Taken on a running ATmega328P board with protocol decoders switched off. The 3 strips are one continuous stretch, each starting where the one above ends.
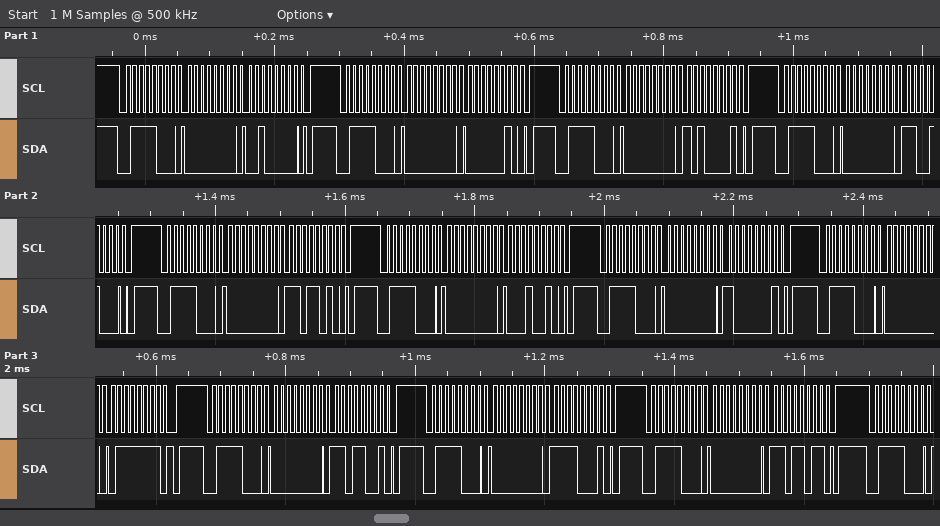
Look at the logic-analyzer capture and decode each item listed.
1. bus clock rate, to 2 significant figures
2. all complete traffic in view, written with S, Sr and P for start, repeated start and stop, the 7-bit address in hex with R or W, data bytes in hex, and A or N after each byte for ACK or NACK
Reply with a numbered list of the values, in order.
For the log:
1. 100 kHz
2. S 3CW A 00 A 20 A P S 3CW A 00 A 02 A P S 3CW A 00 A A1 A P S 3CW A 00 A C8 A P S 3CW A 00 A DA A P S 3CW A 00 A 12 A P S 3CW A 00 A 81 A P S 3CW A 00 A 7F A P S 3CW A 00 A D9 A P S 3CW A 00 A F1 A P S 3CW A 00 A DB A P S 3CW A
